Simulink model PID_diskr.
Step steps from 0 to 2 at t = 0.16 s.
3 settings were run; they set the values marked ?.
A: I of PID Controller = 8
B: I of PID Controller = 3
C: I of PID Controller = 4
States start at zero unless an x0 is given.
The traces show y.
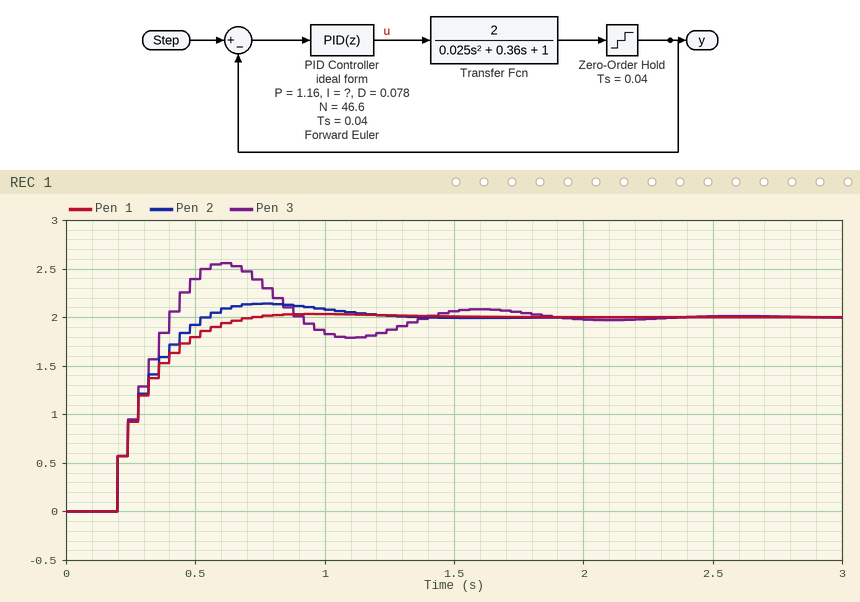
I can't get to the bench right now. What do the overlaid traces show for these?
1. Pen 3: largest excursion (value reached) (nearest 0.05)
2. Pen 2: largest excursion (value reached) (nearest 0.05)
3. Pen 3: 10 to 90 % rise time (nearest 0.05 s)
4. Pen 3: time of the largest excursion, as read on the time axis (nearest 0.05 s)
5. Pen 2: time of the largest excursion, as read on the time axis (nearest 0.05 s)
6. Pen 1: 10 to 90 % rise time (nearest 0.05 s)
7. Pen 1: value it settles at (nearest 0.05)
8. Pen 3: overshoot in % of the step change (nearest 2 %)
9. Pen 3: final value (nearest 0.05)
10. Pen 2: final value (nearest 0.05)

2.55
2.15
0.15 s
0.60 s
0.75 s
0.30 s
2.00
28 %
2.00
2.00
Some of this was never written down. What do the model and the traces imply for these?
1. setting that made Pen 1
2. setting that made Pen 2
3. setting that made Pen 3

B
C
A
